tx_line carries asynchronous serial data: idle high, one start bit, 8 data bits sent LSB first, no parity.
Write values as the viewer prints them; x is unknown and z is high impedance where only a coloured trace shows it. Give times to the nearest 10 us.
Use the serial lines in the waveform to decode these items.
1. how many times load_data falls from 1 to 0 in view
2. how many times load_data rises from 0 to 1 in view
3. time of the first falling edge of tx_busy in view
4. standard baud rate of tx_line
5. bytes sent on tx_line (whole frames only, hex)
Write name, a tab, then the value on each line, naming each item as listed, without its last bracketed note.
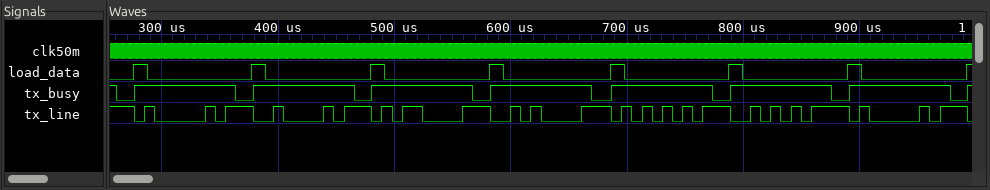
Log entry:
how many times load_data falls from 1 to 0 in view	7
how many times load_data rises from 0 to 1 in view	8
time of the first falling edge of tx_busy in view	260 us
standard baud rate of tx_line	115200 baud
bytes sent on tx_line	41, 42, 0D, 0A, 55, AA, 41
